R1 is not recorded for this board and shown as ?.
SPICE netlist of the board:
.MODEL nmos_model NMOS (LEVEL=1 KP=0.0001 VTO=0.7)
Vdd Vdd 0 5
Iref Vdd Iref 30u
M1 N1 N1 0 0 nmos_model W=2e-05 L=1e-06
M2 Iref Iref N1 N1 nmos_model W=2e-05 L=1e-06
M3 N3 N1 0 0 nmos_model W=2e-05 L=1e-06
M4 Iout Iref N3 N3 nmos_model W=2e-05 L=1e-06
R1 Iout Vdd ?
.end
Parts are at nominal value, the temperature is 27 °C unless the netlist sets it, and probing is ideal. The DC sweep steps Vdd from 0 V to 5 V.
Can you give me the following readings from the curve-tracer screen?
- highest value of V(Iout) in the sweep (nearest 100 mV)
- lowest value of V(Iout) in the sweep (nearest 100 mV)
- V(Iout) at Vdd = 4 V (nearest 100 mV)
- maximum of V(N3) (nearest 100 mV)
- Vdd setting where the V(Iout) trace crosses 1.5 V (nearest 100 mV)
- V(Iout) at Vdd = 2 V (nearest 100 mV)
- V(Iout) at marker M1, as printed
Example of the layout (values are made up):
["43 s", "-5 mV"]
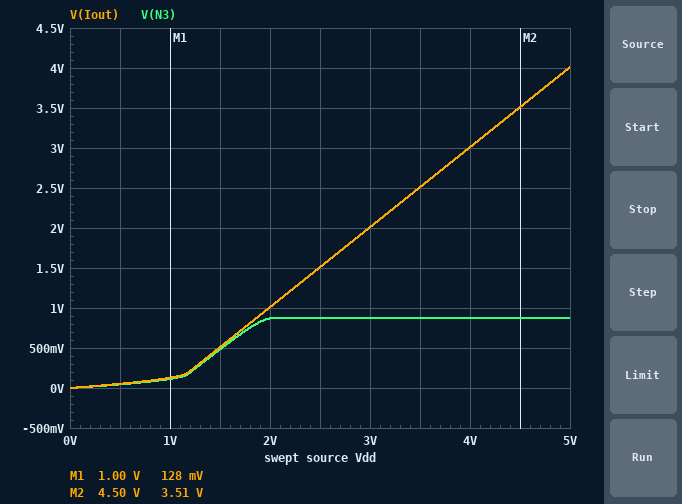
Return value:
["4.0 V", "0 V", "3.0 V", "900 mV", "2.5 V", "1.0 V", "128 mV"]
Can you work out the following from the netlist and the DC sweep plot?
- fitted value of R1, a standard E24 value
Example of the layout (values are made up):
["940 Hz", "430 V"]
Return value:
["33 kΩ"]
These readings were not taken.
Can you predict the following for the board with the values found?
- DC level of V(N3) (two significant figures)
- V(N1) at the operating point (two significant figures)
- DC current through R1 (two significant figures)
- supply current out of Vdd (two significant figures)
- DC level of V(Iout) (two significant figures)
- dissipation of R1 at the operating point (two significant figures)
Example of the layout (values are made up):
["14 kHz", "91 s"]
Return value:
["870 mV", "870 mV", "30 µA", "60 µA", "4.0 V", "30 µW"]
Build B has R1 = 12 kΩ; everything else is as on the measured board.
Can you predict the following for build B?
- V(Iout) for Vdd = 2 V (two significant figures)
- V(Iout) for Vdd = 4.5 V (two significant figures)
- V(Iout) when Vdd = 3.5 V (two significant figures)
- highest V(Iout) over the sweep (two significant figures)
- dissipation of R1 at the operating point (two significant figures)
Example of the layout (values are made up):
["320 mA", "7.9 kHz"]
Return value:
["1.6 V", "4.1 V", "3.1 V", "4.6 V", "11 µW"]
